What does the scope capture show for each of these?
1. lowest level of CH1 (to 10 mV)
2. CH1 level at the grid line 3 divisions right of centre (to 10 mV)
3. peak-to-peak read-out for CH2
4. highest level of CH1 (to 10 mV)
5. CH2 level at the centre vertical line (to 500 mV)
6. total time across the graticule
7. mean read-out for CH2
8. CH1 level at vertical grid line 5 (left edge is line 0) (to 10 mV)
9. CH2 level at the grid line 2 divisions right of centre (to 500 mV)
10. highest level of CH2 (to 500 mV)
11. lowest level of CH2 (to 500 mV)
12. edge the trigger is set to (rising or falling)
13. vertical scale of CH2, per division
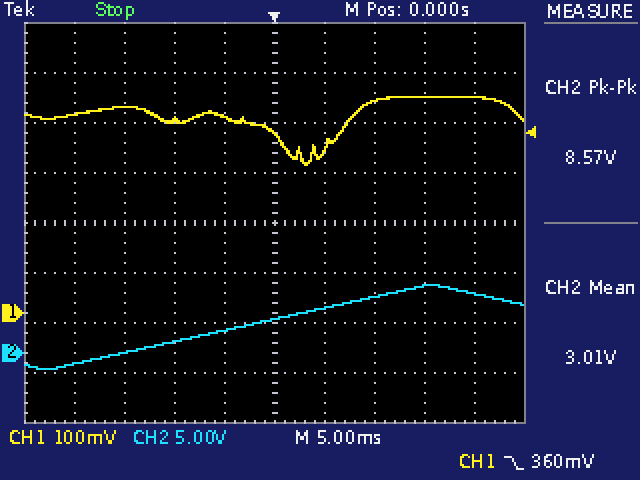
300 mV
430 mV
8.57 V
430 mV
3.5 V
50 ms
3.01 V
360 mV
5.5 V
7.0 V
-1.5 V
falling
5 V
